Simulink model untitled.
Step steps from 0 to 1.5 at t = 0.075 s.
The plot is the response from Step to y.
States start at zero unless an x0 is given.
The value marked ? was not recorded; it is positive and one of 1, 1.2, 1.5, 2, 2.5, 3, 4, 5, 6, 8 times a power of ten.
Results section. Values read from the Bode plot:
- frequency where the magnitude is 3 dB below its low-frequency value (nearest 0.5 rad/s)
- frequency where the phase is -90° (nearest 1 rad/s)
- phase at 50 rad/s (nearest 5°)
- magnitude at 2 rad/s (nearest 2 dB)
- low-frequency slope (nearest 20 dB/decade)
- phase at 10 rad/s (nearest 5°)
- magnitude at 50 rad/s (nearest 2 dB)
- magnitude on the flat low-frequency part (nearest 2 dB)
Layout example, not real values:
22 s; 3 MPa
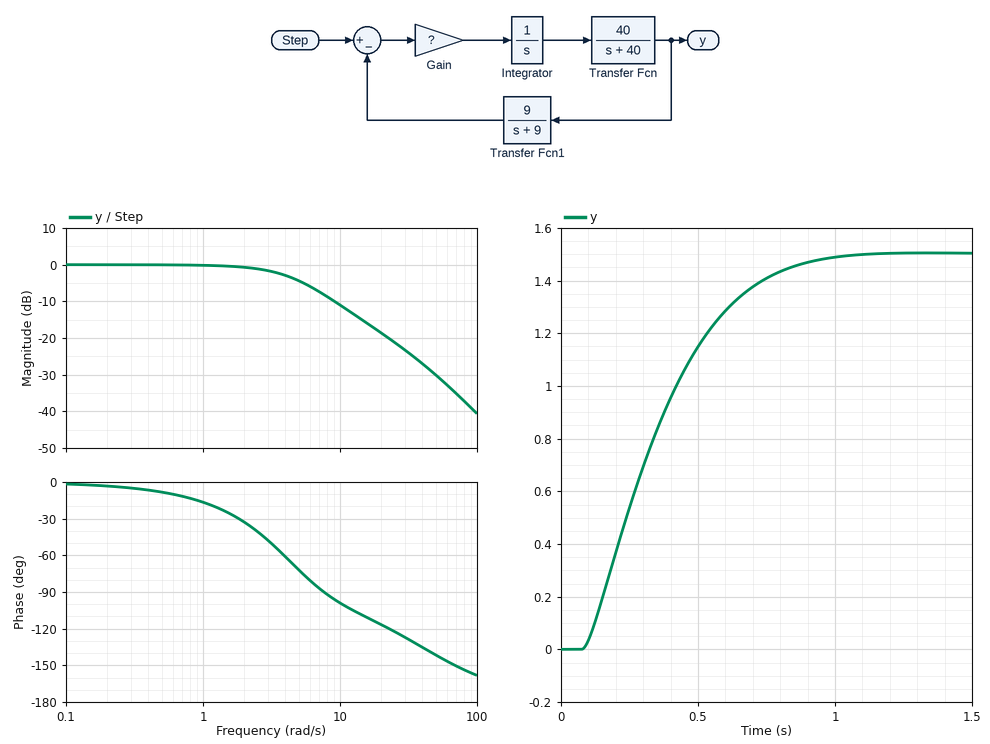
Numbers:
4.0 rad/s; 8 rad/s; -140°; 0 dB; 0 dB/decade; -100°; -30 dB; 0 dB
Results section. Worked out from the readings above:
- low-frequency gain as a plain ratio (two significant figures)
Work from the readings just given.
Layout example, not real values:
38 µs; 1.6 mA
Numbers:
1.0
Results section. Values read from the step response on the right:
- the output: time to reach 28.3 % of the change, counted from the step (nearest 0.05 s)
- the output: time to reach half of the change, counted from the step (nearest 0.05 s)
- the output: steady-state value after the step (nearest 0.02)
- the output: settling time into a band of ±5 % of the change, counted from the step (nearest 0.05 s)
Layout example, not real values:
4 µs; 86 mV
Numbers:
0.15 s; 0.25 s; 1.50; 0.70 s
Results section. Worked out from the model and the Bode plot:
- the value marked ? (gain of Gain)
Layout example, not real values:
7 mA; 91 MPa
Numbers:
2.5
